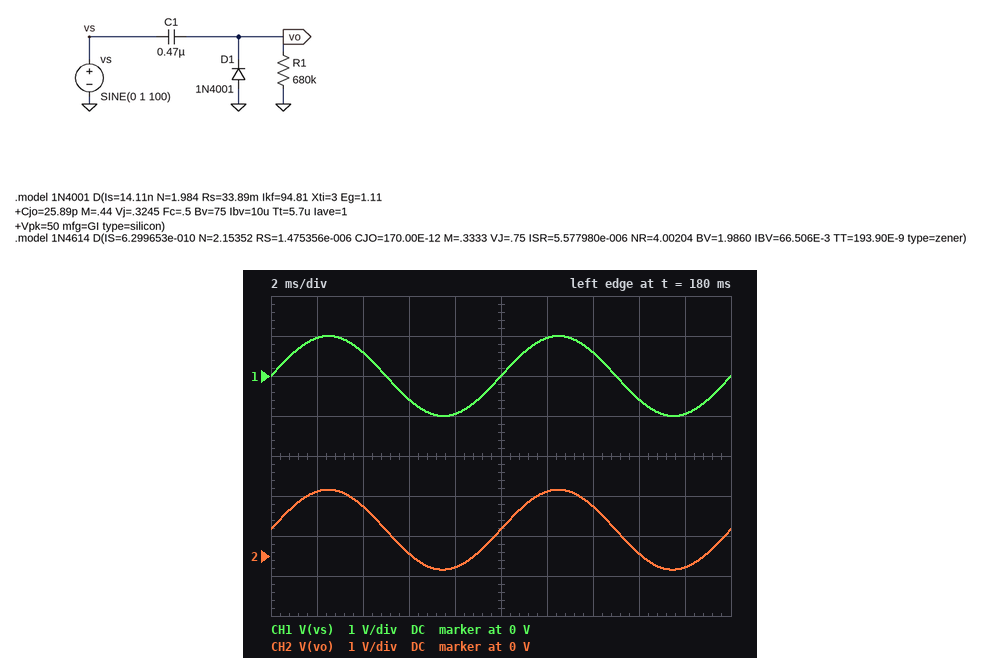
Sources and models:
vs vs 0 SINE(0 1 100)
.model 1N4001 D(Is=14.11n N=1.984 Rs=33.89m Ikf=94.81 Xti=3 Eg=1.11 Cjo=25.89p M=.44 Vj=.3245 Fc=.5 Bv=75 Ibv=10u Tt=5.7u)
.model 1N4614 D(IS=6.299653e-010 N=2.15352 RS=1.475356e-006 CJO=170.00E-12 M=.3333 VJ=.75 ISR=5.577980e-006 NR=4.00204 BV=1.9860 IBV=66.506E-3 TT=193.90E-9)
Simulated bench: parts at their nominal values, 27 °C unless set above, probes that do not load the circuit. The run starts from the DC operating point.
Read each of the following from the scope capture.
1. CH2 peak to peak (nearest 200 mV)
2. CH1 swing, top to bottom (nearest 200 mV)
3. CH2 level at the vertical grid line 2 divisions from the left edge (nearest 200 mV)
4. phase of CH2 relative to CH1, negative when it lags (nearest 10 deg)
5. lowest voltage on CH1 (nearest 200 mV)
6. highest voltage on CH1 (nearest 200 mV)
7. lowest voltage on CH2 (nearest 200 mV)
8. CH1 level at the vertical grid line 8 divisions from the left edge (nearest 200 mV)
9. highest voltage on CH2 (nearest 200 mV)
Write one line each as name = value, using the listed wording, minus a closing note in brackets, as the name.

CH2 peak to peak = 2.0 V
CH1 swing, top to bottom = 2.0 V
CH2 level at the vertical grid line 2 divisions from the left edge = 1.2 V
phase of CH2 relative to CH1, negative when it lags = 0 deg
lowest voltage on CH1 = -1.0 V
highest voltage on CH1 = 1.0 V
lowest voltage on CH2 = -400 mV
CH1 level at the vertical grid line 8 divisions from the left edge = -600 mV
highest voltage on CH2 = 1.6 V
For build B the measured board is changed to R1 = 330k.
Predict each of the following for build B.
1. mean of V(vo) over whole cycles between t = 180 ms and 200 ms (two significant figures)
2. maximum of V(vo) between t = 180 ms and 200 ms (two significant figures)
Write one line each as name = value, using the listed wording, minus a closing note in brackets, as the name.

mean of V(vo) over whole cycles between t = 180 ms and 200 ms = 620 mV
maximum of V(vo) between t = 180 ms and 200 ms = 1.6 V
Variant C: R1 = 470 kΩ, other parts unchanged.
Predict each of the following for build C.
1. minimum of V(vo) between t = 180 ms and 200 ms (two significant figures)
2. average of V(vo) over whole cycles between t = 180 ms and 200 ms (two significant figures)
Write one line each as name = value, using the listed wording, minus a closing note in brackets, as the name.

minimum of V(vo) between t = 180 ms and 200 ms = -360 mV
average of V(vo) over whole cycles between t = 180 ms and 200 ms = 640 mV
